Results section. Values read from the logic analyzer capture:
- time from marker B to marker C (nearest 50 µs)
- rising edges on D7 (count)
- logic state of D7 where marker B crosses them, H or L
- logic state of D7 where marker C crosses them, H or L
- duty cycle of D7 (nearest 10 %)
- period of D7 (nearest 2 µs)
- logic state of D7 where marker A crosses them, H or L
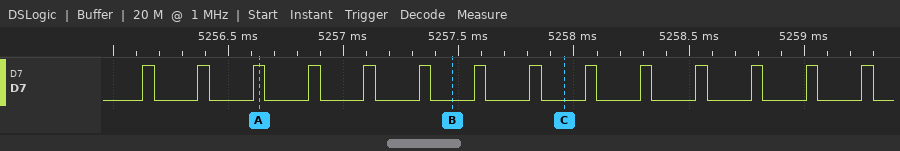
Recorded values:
500 µs
14
D7=L
D7=L
20 %
240 µs
D7=H
